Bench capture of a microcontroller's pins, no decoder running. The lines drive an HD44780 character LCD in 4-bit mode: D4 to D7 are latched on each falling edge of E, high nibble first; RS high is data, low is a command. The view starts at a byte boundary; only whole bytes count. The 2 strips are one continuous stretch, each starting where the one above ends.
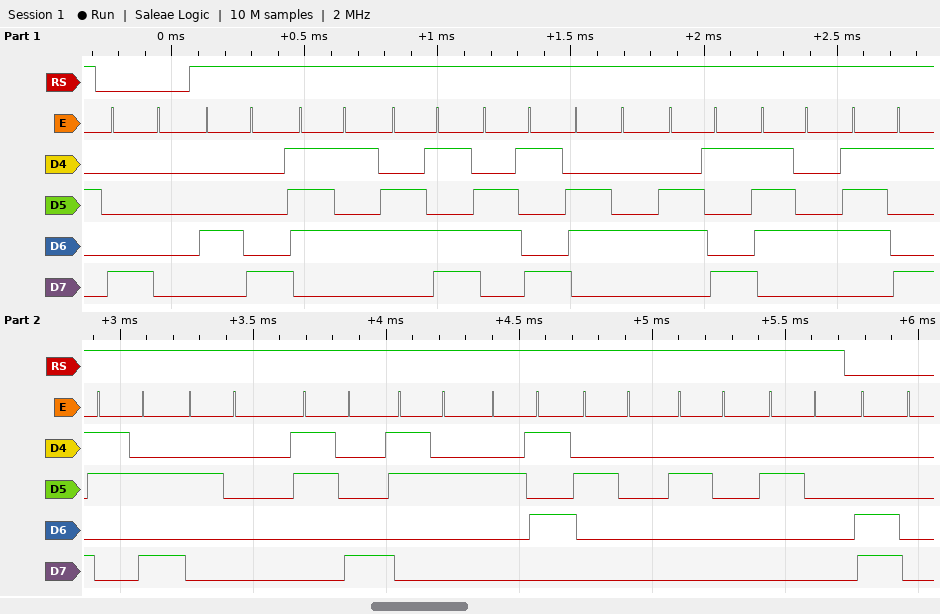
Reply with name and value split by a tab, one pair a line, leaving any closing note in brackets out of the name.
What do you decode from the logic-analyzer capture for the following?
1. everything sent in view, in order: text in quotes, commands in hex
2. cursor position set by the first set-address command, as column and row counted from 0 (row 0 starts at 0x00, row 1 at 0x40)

everything sent in view, in order: text in quotes, commands in hex	0x80 "Humidity: 82%   " 0xC0
cursor position set by the first set-address command, as column and row counted from 0	column 0, row 0
